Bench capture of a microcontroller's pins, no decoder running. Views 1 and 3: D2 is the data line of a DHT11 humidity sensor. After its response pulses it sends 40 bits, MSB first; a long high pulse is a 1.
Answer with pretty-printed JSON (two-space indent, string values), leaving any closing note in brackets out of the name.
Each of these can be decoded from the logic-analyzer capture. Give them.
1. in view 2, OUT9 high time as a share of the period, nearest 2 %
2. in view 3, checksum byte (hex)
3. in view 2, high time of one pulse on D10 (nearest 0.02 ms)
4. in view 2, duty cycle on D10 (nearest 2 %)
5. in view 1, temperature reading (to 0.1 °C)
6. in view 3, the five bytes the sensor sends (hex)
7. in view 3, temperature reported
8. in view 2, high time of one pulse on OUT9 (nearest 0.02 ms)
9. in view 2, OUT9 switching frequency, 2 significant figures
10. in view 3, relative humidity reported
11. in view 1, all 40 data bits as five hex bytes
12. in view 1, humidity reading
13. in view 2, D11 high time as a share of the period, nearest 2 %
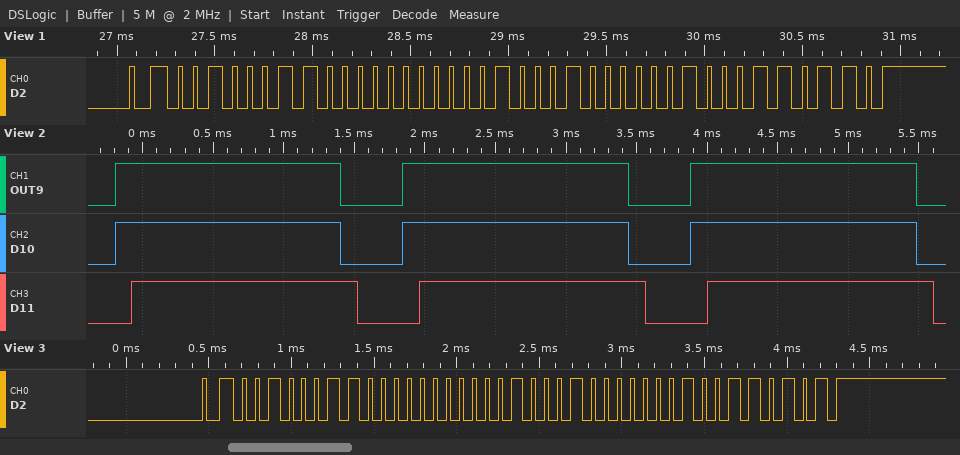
{
  "in view 2, OUT9 high time as a share of the period, nearest 2 %": "78 %",
  "in view 3, checksum byte": "0x35",
  "in view 2, high time of one pulse on D10": "1.60 ms",
  "in view 2, duty cycle on D10": "78 %",
  "in view 1, temperature reading": "17.2 °C",
  "in view 3, the five bytes the sensor sends": "23 00 11 01 35",
  "in view 3, temperature reported": "17.1 °C",
  "in view 2, high time of one pulse on OUT9": "1.60 ms",
  "in view 2, OUT9 switching frequency, 2 significant figures": "490 Hz",
  "in view 3, relative humidity reported": "35 %",
  "in view 1, all 40 data bits as five hex bytes": "23 00 11 02 36",
  "in view 1, humidity reading": "35 %",
  "in view 2, D11 high time as a share of the period, nearest 2 %": "78 %"
}
